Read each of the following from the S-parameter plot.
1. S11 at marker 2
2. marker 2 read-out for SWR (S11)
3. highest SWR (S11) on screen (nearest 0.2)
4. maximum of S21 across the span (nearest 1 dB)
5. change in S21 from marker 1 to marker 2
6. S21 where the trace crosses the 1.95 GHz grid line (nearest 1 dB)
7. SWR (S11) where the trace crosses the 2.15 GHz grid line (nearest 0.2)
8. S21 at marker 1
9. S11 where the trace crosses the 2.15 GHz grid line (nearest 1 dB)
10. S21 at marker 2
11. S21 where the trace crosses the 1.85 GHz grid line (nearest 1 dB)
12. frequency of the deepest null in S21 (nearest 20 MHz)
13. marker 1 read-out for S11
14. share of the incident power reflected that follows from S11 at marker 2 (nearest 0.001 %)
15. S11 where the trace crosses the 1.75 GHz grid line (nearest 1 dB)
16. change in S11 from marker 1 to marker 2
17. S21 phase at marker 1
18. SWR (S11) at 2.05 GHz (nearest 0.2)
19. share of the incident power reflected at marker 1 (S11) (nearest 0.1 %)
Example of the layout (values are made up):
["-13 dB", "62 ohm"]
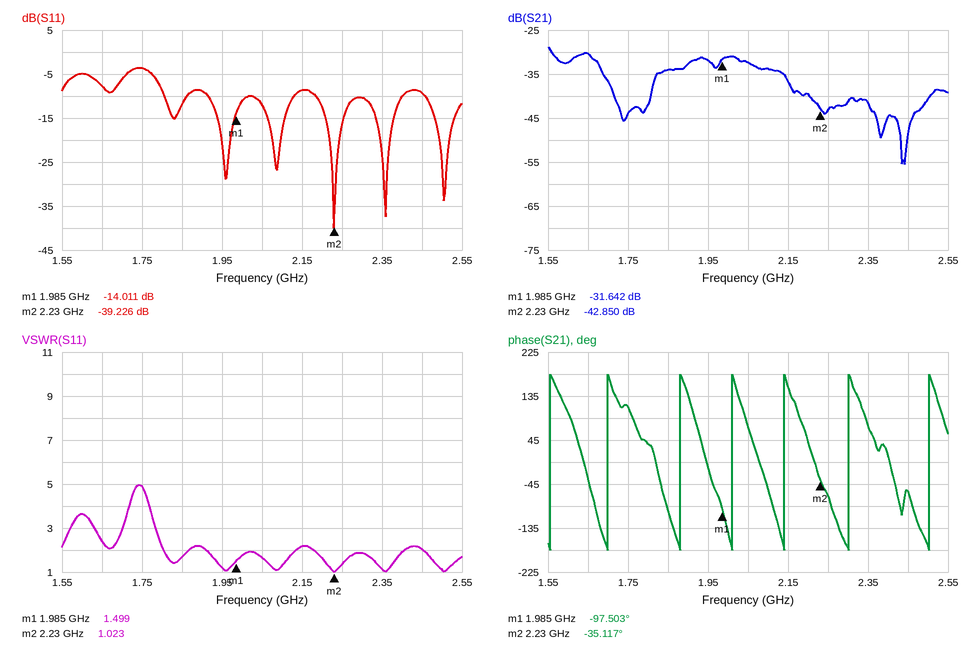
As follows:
["-39.226 dB", "1.023", "5.0", "-29 dB", "-11.208 dB", "-32 dB", "2.2", "-31.642 dB", "-9 dB", "-42.850 dB", "-34 dB", "2.44 GHz", "-14.011 dB", "0.012 %", "-4 dB", "-25.215 dB", "-97.503°", "1.6", "4.0 %"]
